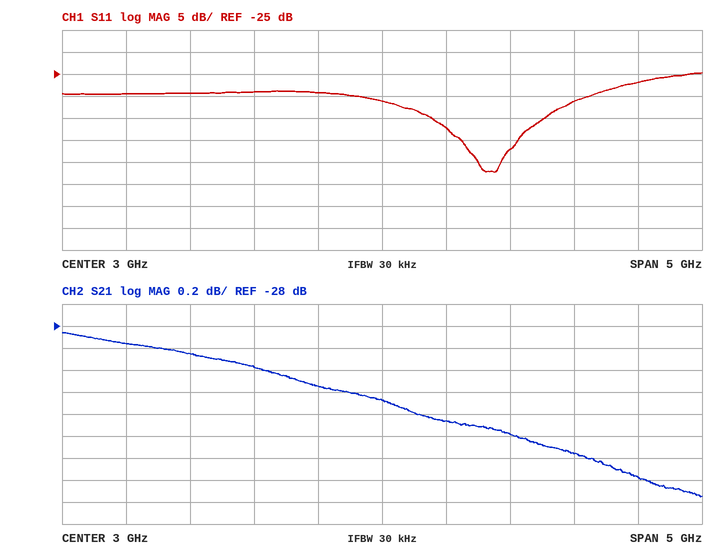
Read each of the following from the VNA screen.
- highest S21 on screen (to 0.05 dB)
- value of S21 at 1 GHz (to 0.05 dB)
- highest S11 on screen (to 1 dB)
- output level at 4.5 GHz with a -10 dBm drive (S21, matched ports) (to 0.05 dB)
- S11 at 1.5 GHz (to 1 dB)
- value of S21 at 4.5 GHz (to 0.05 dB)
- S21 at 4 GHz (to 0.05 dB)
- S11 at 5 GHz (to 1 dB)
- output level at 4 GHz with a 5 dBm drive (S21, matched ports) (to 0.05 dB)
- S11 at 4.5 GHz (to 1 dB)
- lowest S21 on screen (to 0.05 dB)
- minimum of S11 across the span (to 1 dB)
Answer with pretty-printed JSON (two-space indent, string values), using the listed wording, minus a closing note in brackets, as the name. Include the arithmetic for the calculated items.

{
  "highest S21 on screen": "-28.05 dB",
  "value of S21 at 1 GHz": "-28.15 dB",
  "highest S11 on screen": "-25 dB",
  "output level at 4.5 GHz with a -10 dBm drive (S21, matched ports)": "-10 dBm + (-29.15 dB) = -39.15 dBm",
  "S11 at 1.5 GHz": "-29 dB",
  "value of S21 at 4.5 GHz": "-29.15 dB",
  "S21 at 4 GHz": "-29.00 dB",
  "S11 at 5 GHz": "-27 dB",
  "output level at 4 GHz with a 5 dBm drive (S21, matched ports)": "5 dBm + (-29.00 dB) = -24.00 dBm",
  "S11 at 4.5 GHz": "-31 dB",
  "lowest S21 on screen": "-29.55 dB",
  "minimum of S11 across the span": "-47 dB"
}
